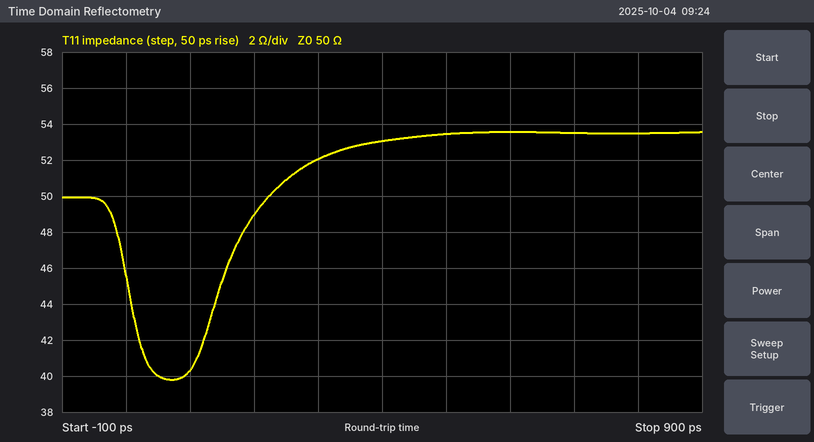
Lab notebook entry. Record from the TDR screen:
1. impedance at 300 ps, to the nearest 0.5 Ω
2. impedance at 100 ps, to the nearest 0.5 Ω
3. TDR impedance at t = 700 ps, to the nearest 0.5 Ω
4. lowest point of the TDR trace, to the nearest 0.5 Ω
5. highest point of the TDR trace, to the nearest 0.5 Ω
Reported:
52.0 Ω
40.5 Ω
53.5 Ω
40.0 Ω
53.5 Ω
